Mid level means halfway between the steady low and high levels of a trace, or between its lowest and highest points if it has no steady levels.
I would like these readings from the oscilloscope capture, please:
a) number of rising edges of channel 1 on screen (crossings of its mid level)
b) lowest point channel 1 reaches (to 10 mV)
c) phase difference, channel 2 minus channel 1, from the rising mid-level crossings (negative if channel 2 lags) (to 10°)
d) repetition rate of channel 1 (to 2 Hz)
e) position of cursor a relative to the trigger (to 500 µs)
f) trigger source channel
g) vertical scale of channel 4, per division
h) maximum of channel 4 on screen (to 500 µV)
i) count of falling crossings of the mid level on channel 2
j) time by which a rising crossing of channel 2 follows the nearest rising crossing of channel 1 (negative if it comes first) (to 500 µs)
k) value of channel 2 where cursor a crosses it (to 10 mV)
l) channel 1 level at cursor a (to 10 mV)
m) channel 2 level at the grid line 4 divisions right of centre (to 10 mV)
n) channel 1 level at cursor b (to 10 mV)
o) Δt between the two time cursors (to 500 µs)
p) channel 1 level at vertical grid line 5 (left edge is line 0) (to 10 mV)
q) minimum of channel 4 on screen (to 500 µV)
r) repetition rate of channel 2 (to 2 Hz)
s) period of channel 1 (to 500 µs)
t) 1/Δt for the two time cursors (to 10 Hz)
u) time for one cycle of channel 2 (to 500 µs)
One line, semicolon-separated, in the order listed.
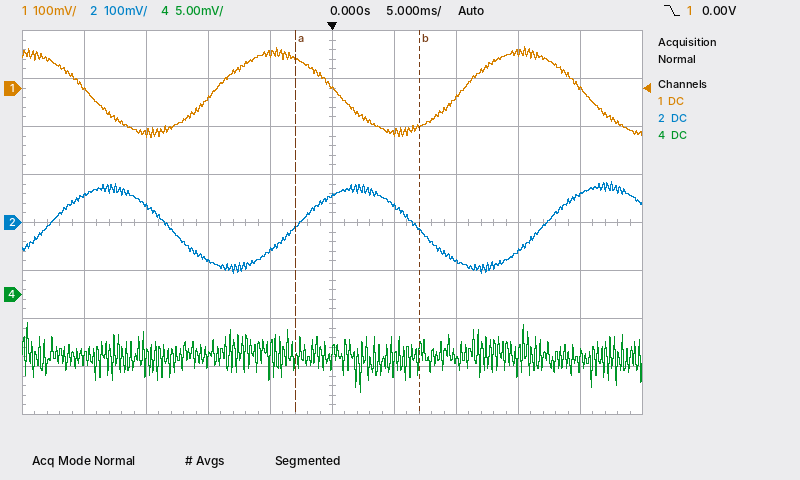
2; -100 mV; -120°; 50 Hz; -3.0 ms; channel 1; 5 mV; -3.0 mV; 2; +6.5 ms; -10 mV; 60 mV; 60 mV; -80 mV; 10.0 ms; 0 mV; -10.0 mV; 50 Hz; 20.0 ms; 100 Hz; 20.0 ms
